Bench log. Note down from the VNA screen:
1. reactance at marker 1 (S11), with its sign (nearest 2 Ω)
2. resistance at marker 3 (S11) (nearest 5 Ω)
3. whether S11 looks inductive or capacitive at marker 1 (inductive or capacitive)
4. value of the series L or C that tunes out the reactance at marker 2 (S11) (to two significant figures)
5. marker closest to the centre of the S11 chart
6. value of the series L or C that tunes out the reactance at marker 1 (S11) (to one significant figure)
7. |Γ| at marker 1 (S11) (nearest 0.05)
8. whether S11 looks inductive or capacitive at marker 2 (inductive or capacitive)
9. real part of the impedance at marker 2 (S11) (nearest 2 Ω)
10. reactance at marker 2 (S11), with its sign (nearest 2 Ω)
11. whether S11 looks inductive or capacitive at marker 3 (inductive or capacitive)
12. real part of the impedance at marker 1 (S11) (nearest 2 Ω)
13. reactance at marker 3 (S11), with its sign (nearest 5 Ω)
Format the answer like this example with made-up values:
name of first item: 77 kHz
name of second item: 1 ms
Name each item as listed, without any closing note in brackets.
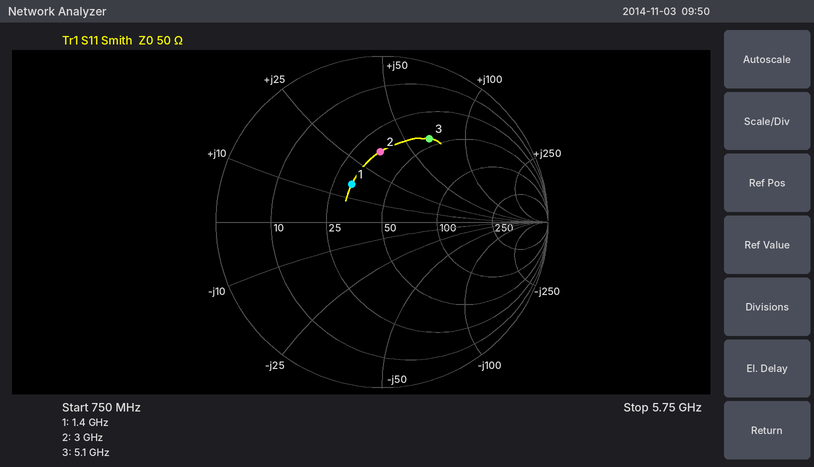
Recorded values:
reactance at marker 1 (S11), with its sign: +16 Ω
resistance at marker 3 (S11): 45 Ω
whether S11 looks inductive or capacitive at marker 1: inductive
value of the series L or C that tunes out the reactance at marker 2 (S11): 1.5 pF
marker closest to the centre of the S11 chart: marker 1
value of the series L or C that tunes out the reactance at marker 1 (S11): 7 pF
|Γ| at marker 1 (S11): 0.30
whether S11 looks inductive or capacitive at marker 2: inductive
real part of the impedance at marker 2 (S11): 34 Ω
reactance at marker 2 (S11), with its sign: +36 Ω
whether S11 looks inductive or capacitive at marker 3: inductive
real part of the impedance at marker 1 (S11): 32 Ω
reactance at marker 3 (S11), with its sign: +65 Ω
